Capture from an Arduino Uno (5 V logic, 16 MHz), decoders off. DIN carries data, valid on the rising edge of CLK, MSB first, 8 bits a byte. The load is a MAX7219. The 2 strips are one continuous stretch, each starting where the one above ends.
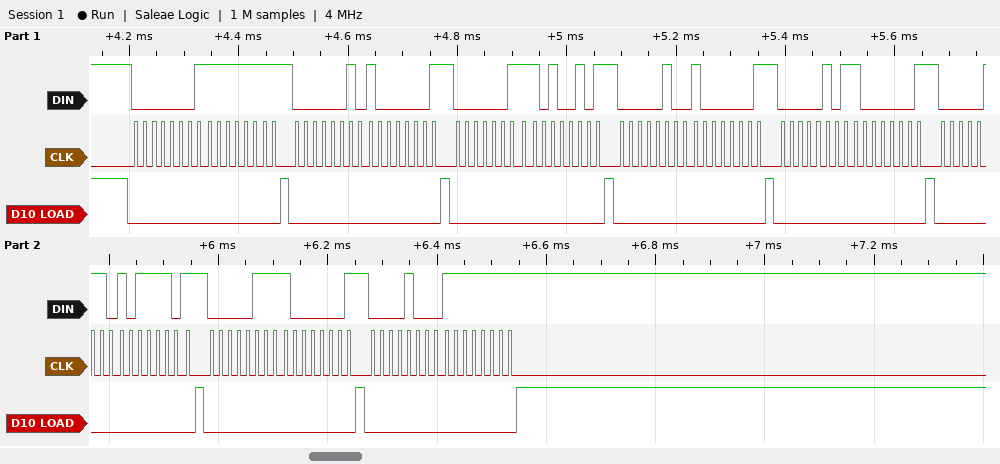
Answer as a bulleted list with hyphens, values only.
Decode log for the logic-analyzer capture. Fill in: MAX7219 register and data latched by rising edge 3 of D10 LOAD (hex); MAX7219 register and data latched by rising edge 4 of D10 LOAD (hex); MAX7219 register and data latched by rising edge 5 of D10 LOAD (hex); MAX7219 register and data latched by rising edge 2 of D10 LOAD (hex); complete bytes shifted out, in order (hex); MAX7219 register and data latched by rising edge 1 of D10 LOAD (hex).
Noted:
- register 0x3, data 0xA5
- register 0x4, data 0x81
- register 0x5, data 0x81
- register 0x2, data 0x81
- 01 FF 02 81 03 A5 04 81 05 81 06 BD 07 81 08 FF
- register 0x1, data 0xFF
